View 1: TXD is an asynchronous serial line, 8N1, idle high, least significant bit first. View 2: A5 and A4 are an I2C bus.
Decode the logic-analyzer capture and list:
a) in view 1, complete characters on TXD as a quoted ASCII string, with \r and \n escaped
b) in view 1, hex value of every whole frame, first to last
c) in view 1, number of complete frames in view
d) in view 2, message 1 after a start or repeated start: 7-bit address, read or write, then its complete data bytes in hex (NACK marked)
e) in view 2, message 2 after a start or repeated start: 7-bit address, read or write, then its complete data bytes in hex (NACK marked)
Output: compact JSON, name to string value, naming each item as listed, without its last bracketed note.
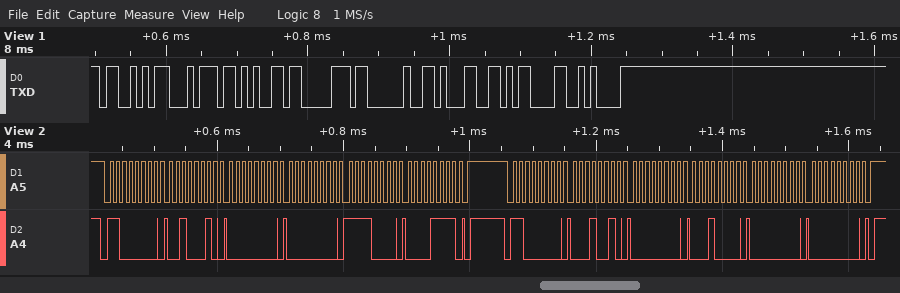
{"in view 1, complete characters on TXD as a quoted ASCII string, with \\r and \\n escaped": "\"Step 1\\r\\n\"", "in view 1, hex value of every whole frame, first to last": "0x53 0x74 0x65 0x70 0x20 0x31 0x0D 0x0A", "in view 1, number of complete frames in view": "8", "in view 2, message 1 after a start or repeated start: 7-bit address, read or write, then its complete data bytes in hex": "0x60 write: 22 00 00 F0 0F", "in view 2, message 2 after a start or repeated start: 7-bit address, read or write, then its complete data bytes in hex": "0x60 write: 12 00 10 00 00"}
